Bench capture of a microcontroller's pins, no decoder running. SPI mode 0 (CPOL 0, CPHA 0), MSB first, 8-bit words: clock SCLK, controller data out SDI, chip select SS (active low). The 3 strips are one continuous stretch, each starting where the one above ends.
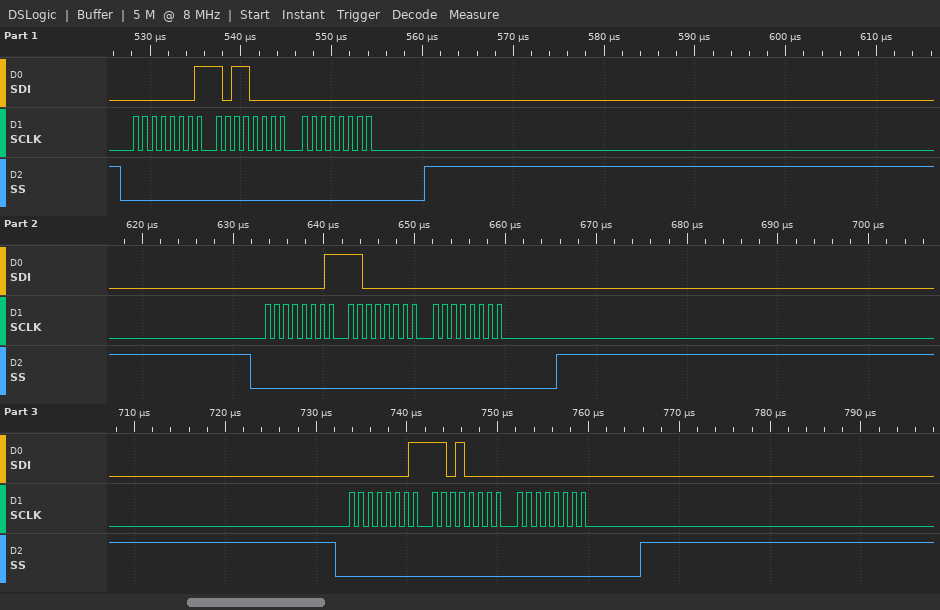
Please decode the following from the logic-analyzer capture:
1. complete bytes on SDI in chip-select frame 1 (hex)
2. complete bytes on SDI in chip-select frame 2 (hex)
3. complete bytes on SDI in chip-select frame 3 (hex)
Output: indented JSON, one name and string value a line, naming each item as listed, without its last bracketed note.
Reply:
{
  "complete bytes on SDI in chip-select frame 1": "01 B0 00",
  "complete bytes on SDI in chip-select frame 2": "01 C0 00",
  "complete bytes on SDI in chip-select frame 3": "01 D0 00"
}
